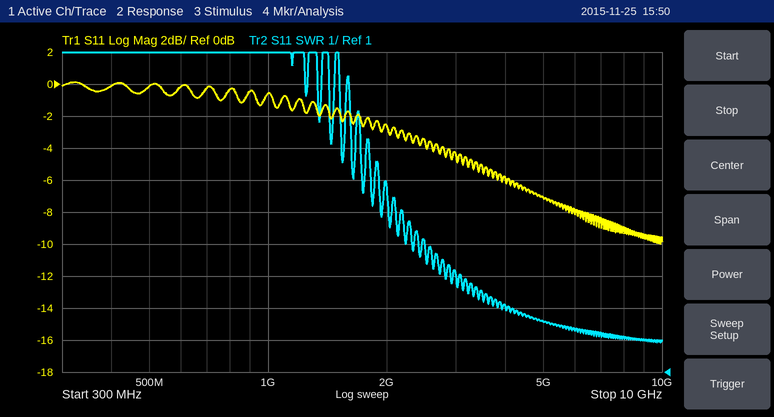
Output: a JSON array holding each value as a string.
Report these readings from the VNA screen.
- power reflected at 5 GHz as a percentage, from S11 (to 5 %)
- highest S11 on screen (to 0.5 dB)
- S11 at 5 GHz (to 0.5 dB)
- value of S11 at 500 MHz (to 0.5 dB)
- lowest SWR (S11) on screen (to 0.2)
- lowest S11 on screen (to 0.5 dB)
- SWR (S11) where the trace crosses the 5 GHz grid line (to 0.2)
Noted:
["20 %", "0.0 dB", "-7.0 dB", "0.0 dB", "2.0", "-10.0 dB", "2.6"]
